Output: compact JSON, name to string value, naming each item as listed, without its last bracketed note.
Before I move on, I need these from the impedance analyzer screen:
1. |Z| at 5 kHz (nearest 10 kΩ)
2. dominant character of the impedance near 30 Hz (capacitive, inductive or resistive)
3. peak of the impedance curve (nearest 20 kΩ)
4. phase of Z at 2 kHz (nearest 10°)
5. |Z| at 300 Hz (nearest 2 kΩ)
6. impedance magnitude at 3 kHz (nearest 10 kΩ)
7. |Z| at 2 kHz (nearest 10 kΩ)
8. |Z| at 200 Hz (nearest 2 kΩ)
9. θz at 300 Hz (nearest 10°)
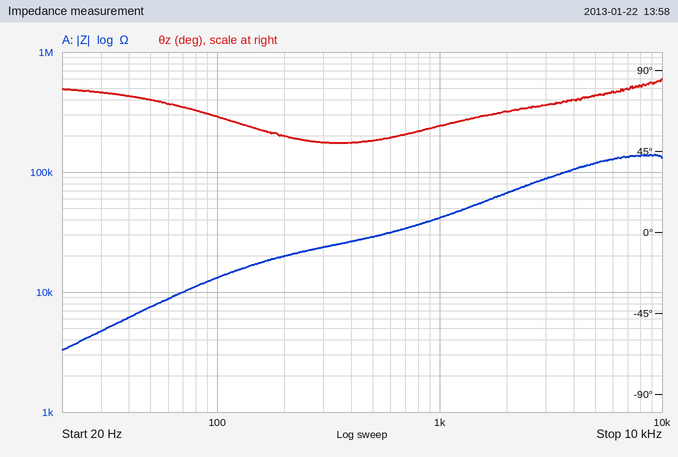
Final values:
{"|Z| at 5 kHz": "120 kΩ", "dominant character of the impedance near 30 Hz": "inductive", "peak of the impedance curve": "140 kΩ", "phase of Z at 2 kHz": "70°", "|Z| at 300 Hz": "24 kΩ", "impedance magnitude at 3 kHz": "90 kΩ", "|Z| at 2 kHz": "70 kΩ", "|Z| at 200 Hz": "20 kΩ", "θz at 300 Hz": "50°"}
